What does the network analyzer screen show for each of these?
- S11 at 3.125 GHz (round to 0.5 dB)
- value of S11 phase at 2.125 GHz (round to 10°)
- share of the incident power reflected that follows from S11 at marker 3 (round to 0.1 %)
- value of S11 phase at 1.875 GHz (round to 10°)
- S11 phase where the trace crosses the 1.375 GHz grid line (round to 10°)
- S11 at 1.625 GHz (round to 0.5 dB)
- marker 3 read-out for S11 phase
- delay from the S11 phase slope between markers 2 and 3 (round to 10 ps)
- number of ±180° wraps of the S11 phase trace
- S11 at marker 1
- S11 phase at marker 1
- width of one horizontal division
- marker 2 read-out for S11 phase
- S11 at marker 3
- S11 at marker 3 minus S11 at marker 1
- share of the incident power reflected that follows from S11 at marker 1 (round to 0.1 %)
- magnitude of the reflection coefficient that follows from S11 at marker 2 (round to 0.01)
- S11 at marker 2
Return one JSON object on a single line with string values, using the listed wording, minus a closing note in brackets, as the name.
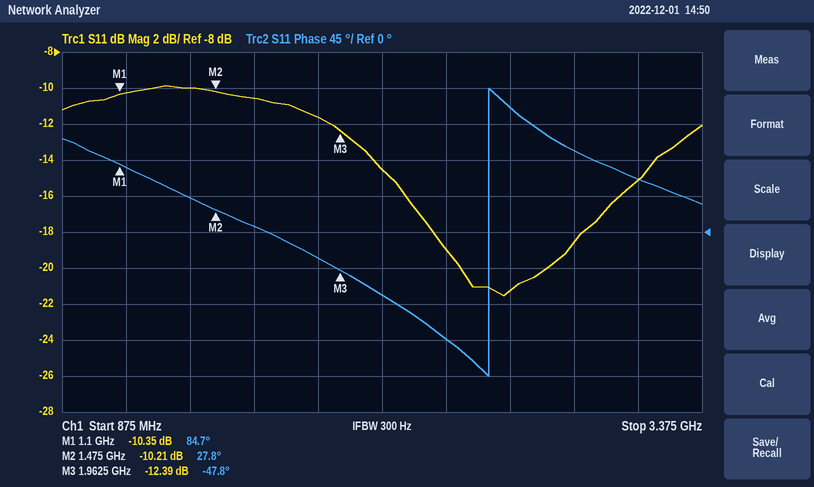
{"S11 at 3.125 GHz": "-15.0 dB", "value of S11 phase at 2.125 GHz": "-80°", "share of the incident power reflected that follows from S11 at marker 3": "5.8 %", "value of S11 phase at 1.875 GHz": "-30°", "S11 phase where the trace crosses the 1.375 GHz grid line": "40°", "S11 at 1.625 GHz": "-10.5 dB", "marker 3 read-out for S11 phase": "-47.8°", "delay from the S11 phase slope between markers 2 and 3": "430 ps", "number of ±180° wraps of the S11 phase trace": "1", "S11 at marker 1": "-10.35 dB", "S11 phase at marker 1": "84.7°", "width of one horizontal division": "250 MHz", "marker 2 read-out for S11 phase": "27.8°", "S11 at marker 3": "-12.39 dB", "S11 at marker 3 minus S11 at marker 1": "-2.04 dB", "share of the incident power reflected that follows from S11 at marker 1": "9.2 %", "magnitude of the reflection coefficient that follows from S11 at marker 2": "0.31", "S11 at marker 2": "-10.21 dB"}
